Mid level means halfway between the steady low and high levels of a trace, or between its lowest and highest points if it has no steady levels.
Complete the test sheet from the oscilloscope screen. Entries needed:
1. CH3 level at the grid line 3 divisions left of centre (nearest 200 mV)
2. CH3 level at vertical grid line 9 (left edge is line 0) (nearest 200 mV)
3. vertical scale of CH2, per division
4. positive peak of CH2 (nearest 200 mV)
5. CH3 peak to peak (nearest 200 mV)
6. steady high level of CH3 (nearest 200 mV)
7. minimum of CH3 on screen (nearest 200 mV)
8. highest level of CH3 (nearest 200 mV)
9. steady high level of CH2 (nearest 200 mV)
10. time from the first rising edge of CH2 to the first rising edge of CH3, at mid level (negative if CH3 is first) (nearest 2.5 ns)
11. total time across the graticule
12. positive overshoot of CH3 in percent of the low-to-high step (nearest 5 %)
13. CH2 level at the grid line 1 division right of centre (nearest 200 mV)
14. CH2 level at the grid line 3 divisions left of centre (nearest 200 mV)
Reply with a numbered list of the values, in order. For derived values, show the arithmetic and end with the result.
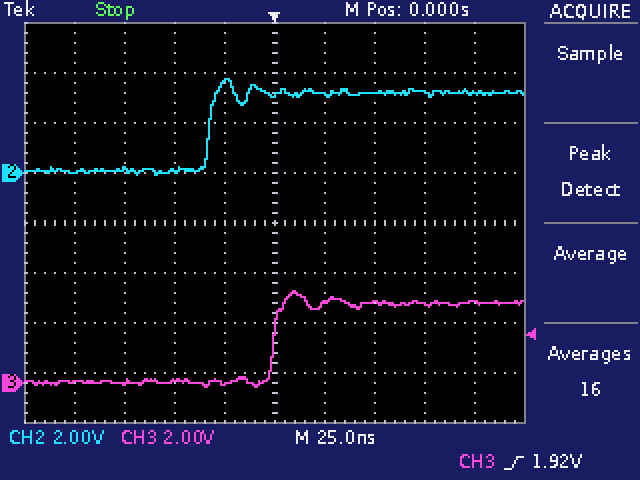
1. 0.0 V
2. 3.2 V
3. 2 V
4. 3.8 V
5. 3.6 V − (-200 mV) = 3.8 V
6. 3.2 V
7. -200 mV
8. 3.6 V
9. 3.2 V
10. +32.5 ns
11. 250 ns
12. 15 %
13. 3.2 V
14. 200 mV
